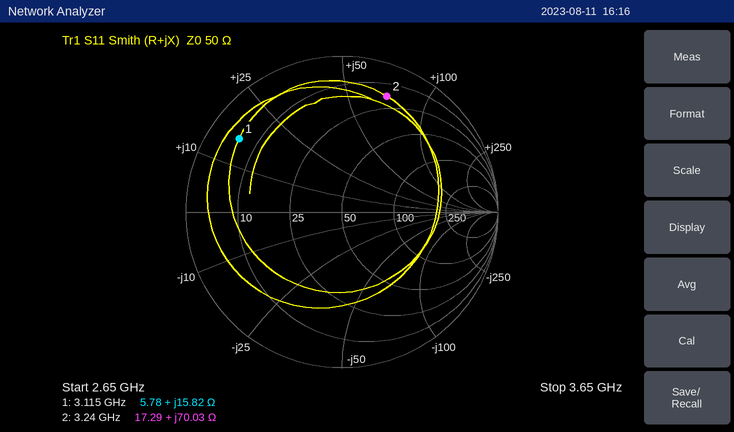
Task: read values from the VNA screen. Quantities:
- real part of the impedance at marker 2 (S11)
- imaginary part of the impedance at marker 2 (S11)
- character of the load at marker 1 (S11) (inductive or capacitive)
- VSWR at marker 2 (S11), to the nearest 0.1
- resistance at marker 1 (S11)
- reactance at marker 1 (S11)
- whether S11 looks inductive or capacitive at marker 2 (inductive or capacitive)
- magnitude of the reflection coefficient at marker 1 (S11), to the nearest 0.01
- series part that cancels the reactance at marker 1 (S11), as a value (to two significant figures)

17.29 Ω
+70.03 Ω
inductive
8.8
5.78 Ω
+15.82 Ω
inductive
0.81
3.2 pF
